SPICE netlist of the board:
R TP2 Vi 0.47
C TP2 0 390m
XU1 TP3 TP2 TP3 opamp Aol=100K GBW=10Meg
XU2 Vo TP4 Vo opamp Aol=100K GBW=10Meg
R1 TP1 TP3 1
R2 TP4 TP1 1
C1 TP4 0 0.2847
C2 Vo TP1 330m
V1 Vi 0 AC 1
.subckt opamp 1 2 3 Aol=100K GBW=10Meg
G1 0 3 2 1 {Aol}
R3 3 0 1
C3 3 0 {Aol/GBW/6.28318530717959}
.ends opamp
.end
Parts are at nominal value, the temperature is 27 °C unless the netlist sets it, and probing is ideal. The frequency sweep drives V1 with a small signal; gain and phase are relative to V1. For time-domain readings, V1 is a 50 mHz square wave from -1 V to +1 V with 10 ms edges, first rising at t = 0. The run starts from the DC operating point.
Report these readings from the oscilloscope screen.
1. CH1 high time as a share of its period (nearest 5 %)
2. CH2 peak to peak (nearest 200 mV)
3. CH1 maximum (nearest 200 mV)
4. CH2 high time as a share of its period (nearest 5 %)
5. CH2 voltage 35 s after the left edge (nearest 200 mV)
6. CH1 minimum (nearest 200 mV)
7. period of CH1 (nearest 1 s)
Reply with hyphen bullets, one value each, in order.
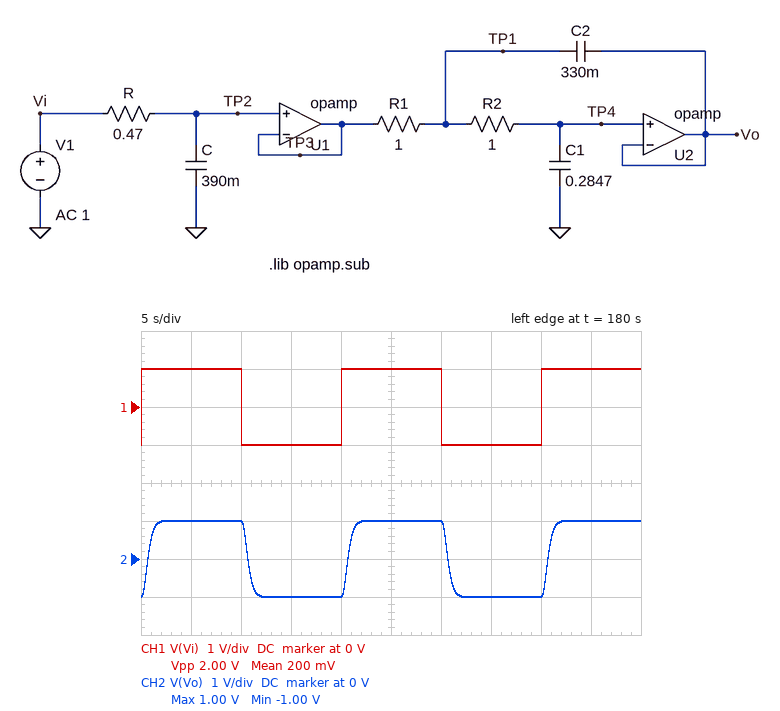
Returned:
- 50 %
- 2.0 V
- 1.0 V
- 50 %
- -1.0 V
- -1.0 V
- 20 s
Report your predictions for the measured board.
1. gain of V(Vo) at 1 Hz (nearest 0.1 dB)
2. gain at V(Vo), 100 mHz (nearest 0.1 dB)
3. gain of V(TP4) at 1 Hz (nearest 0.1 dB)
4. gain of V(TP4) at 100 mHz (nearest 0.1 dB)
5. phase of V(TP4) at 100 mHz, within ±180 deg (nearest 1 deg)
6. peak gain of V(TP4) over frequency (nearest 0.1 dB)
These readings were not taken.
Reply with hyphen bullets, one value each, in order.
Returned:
- -16.7 dB
- -0.3 dB
- -16.7 dB
- -0.3 dB
- -27 deg
- 0 dB
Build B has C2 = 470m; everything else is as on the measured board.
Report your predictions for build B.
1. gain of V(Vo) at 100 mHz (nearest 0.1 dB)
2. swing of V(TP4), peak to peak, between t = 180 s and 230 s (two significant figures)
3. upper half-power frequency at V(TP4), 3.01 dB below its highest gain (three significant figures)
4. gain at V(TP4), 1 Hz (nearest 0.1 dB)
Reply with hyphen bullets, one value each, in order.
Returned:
- -0.2 dB
- 2.1 V
- 354 mHz
- -18.6 dB
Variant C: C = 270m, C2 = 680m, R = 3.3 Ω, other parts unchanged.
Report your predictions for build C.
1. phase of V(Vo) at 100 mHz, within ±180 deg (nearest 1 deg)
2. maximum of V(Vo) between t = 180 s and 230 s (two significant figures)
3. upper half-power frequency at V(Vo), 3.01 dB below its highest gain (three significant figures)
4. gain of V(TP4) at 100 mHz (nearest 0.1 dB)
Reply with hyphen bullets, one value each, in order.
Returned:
- -50 deg
- 1.0 V
- 182 mHz
- -1.1 dB
